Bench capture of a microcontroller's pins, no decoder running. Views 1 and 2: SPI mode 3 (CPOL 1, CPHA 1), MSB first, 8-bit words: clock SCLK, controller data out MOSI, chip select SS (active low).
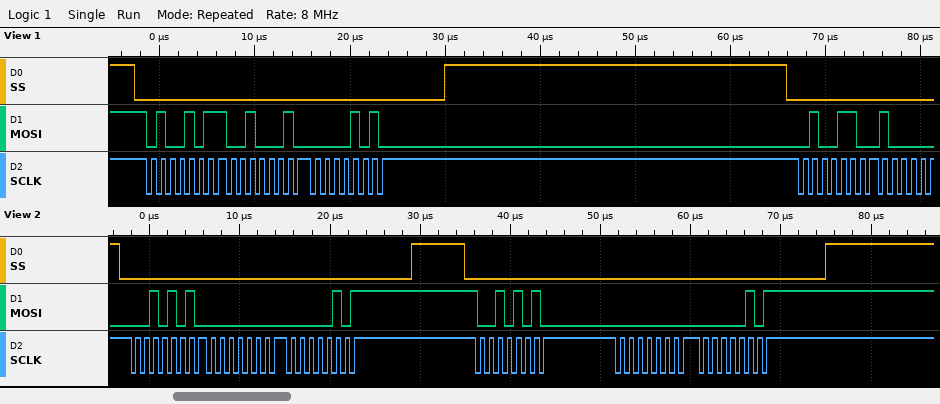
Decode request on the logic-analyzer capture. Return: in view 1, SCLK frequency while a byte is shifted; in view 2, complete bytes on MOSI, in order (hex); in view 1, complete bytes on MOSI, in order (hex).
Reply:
1 MHz
2A 00 05 2A 00 05
4B 22 0A 4C
